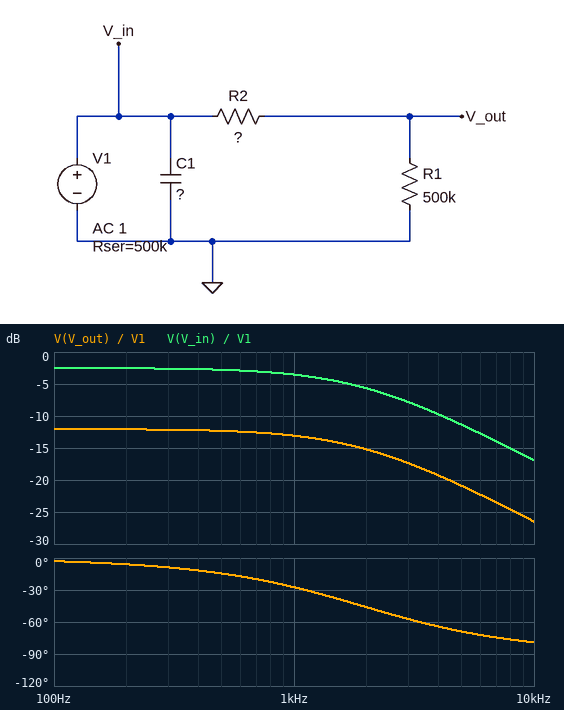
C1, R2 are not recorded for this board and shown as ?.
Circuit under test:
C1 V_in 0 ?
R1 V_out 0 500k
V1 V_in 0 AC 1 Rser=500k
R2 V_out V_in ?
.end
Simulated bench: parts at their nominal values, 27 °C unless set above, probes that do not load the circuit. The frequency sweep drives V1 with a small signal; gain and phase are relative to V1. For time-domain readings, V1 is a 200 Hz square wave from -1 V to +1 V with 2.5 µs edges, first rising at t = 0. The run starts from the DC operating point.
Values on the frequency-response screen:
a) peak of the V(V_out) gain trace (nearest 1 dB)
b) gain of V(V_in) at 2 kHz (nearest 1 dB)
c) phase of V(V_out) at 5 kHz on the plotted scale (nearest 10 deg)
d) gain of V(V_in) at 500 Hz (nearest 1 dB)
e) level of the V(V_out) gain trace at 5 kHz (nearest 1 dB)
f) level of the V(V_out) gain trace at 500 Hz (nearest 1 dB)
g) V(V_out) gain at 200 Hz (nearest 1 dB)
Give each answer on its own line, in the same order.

-12 dB
-6 dB
-70 deg
-3 dB
-21 dB
-12 dB
-12 dB
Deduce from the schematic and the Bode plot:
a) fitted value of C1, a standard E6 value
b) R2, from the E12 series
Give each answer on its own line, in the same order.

220 pF
1 MΩ
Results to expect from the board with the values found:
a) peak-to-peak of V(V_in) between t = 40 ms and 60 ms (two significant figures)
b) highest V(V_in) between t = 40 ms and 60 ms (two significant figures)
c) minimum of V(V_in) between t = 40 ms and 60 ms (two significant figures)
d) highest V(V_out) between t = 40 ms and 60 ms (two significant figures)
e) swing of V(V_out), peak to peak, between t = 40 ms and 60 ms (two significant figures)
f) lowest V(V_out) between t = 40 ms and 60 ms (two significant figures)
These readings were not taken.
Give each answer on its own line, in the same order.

1.5 V
750 mV
-750 mV
250 mV
500 mV
-250 mV
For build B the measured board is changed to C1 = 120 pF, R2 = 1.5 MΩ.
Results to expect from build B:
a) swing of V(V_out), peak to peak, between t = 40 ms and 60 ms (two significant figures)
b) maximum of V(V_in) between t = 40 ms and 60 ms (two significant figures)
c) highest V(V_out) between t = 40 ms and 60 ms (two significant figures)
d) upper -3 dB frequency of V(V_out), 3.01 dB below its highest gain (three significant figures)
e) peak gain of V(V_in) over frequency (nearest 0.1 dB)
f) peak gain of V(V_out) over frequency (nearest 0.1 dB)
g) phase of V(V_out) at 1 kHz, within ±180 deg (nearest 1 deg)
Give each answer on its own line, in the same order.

400 mV
800 mV
200 mV
3.32 kHz
-1.9 dB
-14.0 dB
-17 deg
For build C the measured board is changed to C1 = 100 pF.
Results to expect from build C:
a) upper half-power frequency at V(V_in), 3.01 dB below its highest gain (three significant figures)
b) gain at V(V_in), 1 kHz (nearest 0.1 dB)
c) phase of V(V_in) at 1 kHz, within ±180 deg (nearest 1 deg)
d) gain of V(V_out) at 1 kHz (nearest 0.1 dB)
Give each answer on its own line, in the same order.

4.24 kHz
-2.7 dB
-13 deg
-12.3 dB
